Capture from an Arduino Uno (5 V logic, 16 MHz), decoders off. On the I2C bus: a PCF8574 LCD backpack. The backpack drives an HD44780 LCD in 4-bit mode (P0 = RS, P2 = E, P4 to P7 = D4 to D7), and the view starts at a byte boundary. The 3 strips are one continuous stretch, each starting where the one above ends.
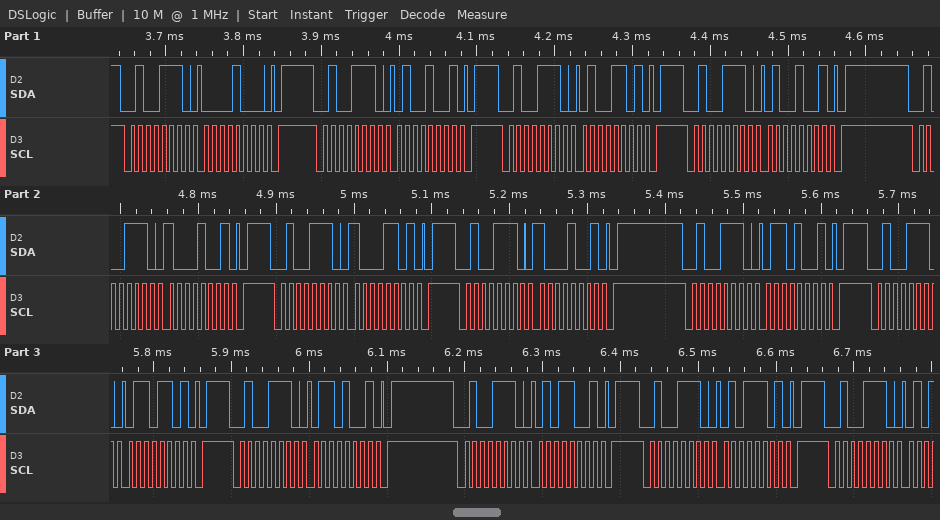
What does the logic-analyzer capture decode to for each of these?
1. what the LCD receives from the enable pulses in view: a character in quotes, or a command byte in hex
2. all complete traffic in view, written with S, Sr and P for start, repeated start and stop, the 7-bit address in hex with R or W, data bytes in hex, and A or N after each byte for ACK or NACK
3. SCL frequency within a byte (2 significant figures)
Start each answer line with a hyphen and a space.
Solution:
- 'H'
- S 27W A 08 A P S 27W A 49 A P S 27W A 4D A P S 27W A 49 A P S 27W A 89 A P S 27W A 8D A P S 27W A 89 A P S 27W A 69 A P S 27W A 6D A P S 27W A 69 A P S 27W A 59 A P S 27W A 5D A P S 27W A
- 100 kHz
